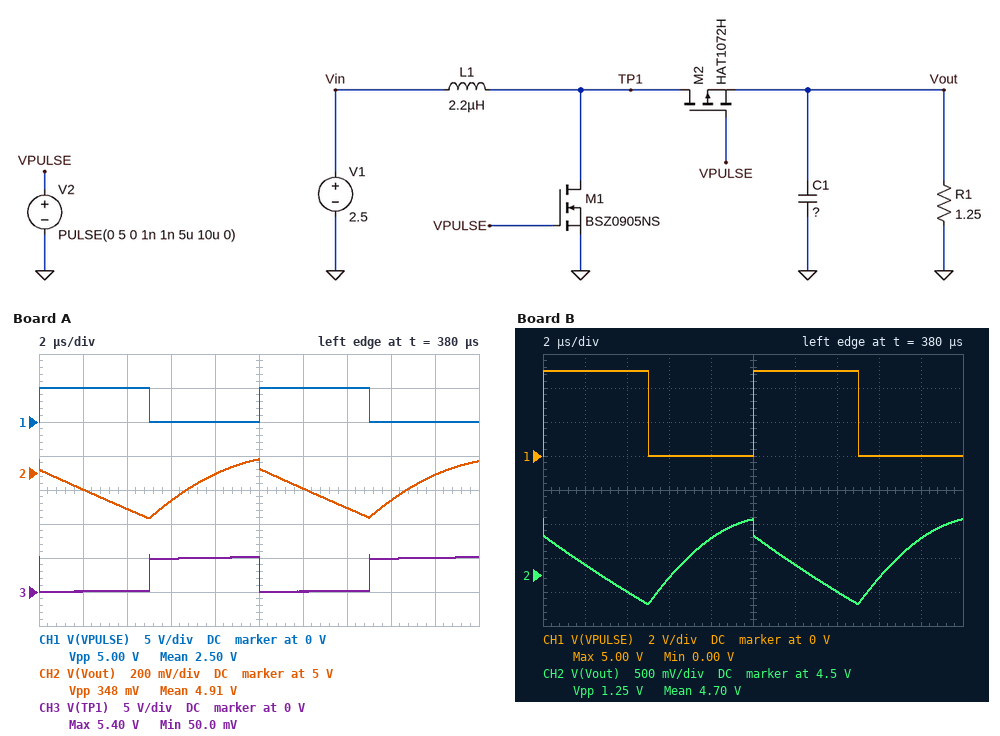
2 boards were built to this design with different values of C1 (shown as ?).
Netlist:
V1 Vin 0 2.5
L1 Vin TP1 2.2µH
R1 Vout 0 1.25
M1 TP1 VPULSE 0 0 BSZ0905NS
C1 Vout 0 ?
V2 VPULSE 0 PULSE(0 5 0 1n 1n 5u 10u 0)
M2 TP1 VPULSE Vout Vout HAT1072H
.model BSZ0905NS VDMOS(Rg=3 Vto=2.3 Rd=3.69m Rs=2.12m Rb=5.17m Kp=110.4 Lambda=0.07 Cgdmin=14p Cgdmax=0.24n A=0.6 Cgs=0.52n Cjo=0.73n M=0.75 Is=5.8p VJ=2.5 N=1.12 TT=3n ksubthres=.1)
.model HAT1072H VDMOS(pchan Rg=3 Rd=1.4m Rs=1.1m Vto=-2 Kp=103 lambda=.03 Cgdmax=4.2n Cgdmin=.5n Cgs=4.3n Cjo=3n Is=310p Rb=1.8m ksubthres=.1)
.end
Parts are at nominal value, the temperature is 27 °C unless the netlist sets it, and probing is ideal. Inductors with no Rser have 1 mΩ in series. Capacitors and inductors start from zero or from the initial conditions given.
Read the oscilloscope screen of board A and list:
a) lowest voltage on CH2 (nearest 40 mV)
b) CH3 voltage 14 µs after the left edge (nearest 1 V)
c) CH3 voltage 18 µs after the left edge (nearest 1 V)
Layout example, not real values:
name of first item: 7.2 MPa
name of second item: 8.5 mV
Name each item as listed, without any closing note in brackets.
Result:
lowest voltage on CH2: 4.72 V
CH3 voltage 14 µs after the left edge: 0 V
CH3 voltage 18 µs after the left edge: 5 V
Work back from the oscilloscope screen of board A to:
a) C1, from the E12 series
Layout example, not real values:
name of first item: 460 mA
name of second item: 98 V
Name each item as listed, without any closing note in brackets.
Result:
C1, from the E12 series: 68 µF
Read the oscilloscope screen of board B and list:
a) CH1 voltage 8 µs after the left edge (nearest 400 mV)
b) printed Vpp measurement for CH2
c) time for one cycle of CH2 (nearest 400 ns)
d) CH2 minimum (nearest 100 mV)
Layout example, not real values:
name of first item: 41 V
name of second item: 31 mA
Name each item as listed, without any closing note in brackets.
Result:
CH1 voltage 8 µs after the left edge: 0 V
printed Vpp measurement for CH2: 1.25 V
time for one cycle of CH2: 10.0 µs
CH2 minimum: 4.1 V
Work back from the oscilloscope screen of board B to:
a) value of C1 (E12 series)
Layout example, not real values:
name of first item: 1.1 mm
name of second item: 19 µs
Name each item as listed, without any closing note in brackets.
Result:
value of C1: 18 µF
